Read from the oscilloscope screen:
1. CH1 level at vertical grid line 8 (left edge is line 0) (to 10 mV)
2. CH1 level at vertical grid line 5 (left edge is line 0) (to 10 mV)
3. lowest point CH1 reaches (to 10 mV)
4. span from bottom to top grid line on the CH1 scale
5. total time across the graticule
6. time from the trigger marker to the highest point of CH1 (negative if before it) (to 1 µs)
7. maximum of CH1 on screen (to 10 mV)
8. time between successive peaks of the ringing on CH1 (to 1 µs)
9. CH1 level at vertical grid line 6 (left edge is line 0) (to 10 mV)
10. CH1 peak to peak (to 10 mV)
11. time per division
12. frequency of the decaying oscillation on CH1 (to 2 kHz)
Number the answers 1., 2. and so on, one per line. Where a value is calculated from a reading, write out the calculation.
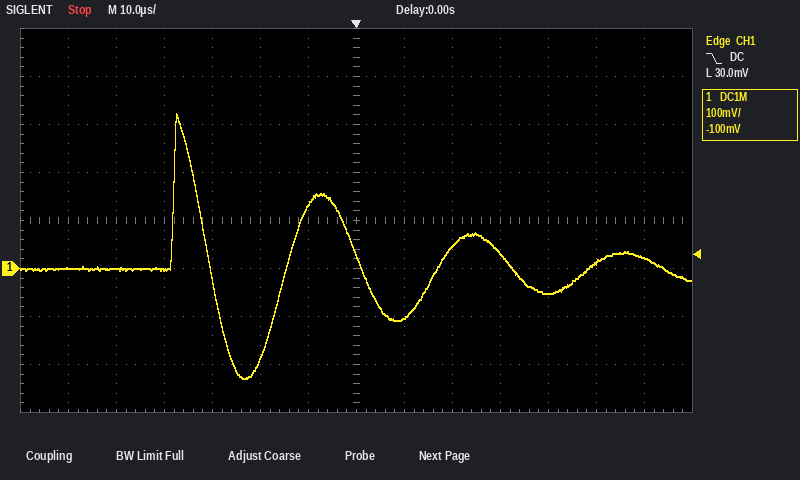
1. -100 mV
2. -190 mV
3. -230 mV
4. 800 mV
5. 140 µs
6. -37 µs
7. 320 mV
8. 31 µs
9. 130 mV
10. 320 mV − (-230 mV) = 550 mV
11. 10 µs
12. 1 / 31 µs ≈ 32 kHz
